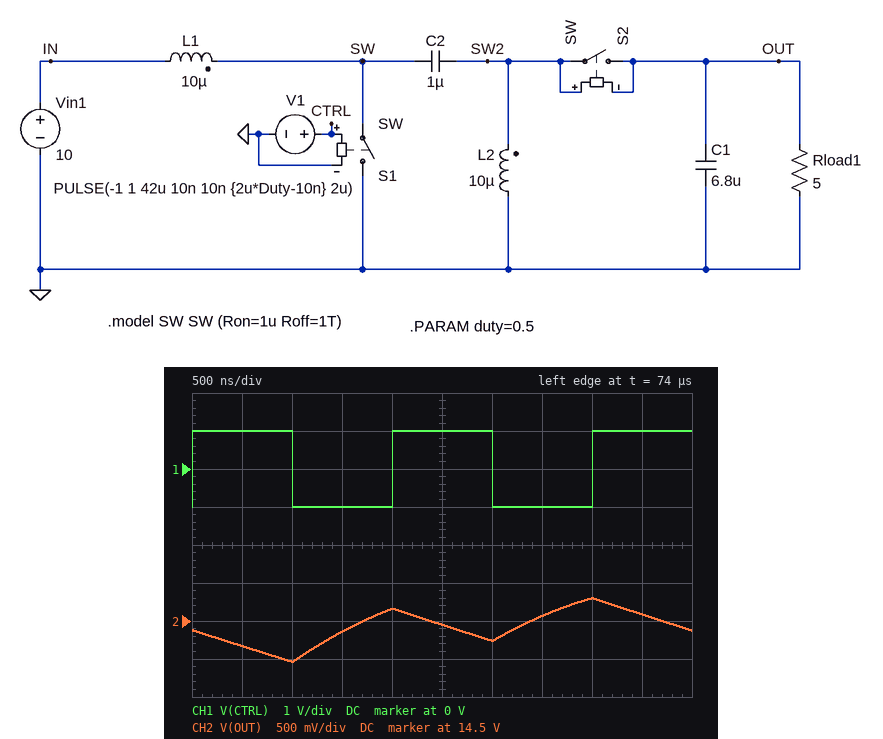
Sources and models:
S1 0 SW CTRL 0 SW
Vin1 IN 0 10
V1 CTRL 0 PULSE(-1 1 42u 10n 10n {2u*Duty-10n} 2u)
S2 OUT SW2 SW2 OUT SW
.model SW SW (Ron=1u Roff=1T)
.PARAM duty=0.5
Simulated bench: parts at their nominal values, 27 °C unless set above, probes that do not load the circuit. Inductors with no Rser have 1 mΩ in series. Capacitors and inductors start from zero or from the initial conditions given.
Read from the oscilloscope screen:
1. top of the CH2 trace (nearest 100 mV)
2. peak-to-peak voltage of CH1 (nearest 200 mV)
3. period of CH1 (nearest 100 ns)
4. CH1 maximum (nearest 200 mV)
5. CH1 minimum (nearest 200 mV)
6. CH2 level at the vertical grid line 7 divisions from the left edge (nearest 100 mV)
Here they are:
14.8 V
2.0 V
2.0 µs
1.0 V
-1.0 V
14.6 V
